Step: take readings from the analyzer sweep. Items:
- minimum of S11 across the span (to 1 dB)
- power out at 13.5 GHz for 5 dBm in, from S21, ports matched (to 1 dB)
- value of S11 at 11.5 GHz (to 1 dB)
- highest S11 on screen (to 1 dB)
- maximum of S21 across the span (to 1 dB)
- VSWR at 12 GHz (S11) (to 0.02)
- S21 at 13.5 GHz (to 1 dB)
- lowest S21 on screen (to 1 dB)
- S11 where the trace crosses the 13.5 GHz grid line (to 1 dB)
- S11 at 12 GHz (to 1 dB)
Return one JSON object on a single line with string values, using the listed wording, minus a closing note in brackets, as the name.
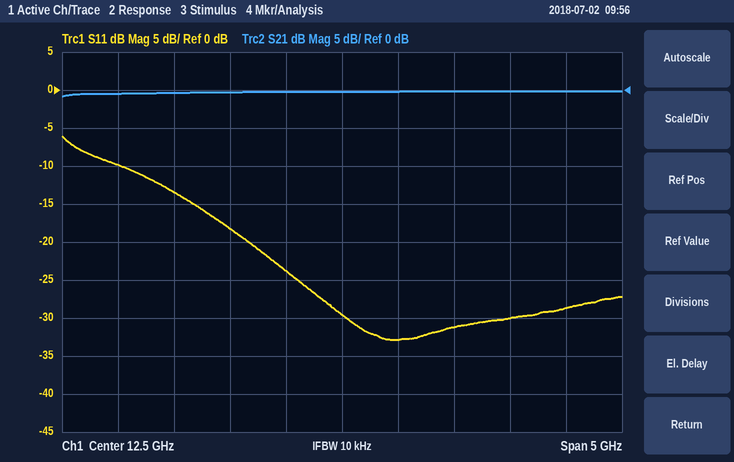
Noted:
{"minimum of S11 across the span": "-33 dB", "power out at 13.5 GHz for 5 dBm in, from S21, ports matched": "5 dBm", "value of S11 at 11.5 GHz": "-18 dB", "highest S11 on screen": "-6 dB", "maximum of S21 across the span": "0 dB", "VSWR at 12 GHz (S11)": "1.14", "S21 at 13.5 GHz": "0 dB", "lowest S21 on screen": "-1 dB", "S11 where the trace crosses the 13.5 GHz grid line": "-31 dB", "S11 at 12 GHz": "-24 dB"}
